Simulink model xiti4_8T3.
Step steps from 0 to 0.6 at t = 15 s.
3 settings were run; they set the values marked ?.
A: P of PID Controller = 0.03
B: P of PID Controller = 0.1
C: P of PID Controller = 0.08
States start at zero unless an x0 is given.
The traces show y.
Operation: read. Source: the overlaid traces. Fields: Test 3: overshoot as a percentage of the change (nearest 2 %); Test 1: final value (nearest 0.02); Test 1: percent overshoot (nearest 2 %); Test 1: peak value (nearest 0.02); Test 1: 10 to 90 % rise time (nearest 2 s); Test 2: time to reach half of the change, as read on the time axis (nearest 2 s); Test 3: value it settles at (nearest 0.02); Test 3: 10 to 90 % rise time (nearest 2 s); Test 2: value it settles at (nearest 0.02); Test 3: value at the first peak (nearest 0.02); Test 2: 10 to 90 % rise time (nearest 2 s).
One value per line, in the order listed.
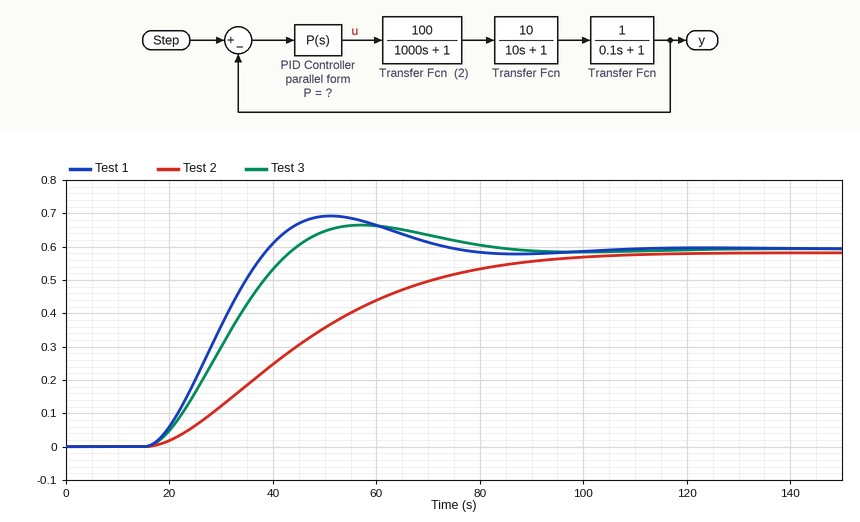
12 %
0.60
16 %
0.70
16 s
44 s
0.60
20 s
0.58
0.66
52 s
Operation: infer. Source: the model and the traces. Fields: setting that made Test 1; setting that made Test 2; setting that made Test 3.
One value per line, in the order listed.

B
A
C
